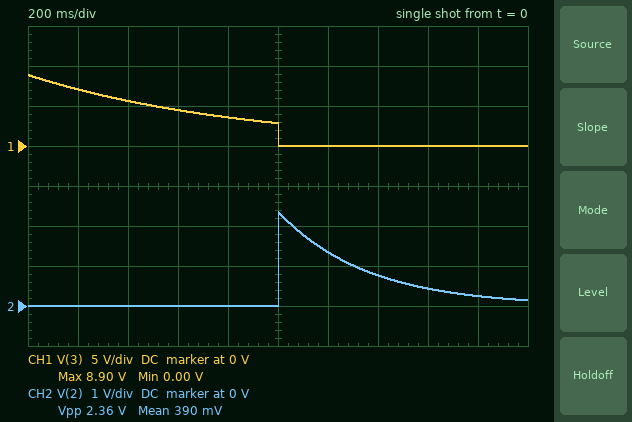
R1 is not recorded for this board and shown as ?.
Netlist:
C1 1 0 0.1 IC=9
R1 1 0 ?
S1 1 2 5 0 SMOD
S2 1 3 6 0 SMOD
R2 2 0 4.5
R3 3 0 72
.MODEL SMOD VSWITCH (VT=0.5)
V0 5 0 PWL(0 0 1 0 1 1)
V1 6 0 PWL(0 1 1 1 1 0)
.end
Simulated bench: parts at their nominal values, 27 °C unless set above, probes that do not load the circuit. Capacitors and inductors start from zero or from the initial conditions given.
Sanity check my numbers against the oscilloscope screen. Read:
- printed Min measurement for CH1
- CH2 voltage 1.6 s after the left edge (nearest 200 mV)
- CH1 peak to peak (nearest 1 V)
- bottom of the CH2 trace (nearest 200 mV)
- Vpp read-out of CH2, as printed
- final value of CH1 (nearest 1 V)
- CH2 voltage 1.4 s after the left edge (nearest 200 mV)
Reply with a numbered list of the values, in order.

1. 0.00 V
2. 400 mV
3. 9 V
4. 0 V
5. 2.36 V
6. 0 V
7. 800 mV
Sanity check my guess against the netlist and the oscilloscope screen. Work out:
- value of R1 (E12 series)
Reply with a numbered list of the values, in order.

1. 10 Ω
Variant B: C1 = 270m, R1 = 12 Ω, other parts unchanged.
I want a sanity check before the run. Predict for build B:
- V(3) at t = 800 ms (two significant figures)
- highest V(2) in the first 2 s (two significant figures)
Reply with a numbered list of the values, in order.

1. 6.7 V
2. 5.1 V
